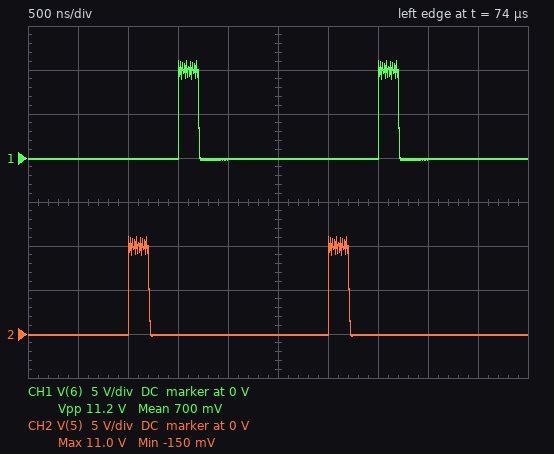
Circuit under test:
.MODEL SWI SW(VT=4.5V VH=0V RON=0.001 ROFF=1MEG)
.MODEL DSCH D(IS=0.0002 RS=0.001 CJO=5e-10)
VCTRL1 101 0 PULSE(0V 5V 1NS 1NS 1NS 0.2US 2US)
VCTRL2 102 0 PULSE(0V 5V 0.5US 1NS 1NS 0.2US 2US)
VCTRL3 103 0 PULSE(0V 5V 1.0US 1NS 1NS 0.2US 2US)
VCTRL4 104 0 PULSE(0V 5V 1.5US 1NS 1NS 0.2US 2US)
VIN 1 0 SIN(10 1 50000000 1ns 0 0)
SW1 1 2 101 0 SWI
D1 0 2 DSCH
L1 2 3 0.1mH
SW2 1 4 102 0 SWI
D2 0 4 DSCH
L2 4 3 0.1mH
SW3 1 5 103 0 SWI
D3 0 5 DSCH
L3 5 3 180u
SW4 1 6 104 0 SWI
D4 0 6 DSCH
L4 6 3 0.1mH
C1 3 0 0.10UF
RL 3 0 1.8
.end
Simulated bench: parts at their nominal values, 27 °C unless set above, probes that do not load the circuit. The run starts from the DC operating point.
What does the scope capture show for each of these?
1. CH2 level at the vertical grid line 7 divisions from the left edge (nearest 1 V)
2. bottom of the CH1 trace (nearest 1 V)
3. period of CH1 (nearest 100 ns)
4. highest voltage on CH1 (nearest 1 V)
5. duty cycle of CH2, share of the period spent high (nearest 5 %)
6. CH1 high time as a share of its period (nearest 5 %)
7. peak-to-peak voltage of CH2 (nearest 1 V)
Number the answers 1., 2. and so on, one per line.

1. 0 V
2. 0 V
3. 2.0 µs
4. 11 V
5. 10 %
6. 10 %
7. 11 V
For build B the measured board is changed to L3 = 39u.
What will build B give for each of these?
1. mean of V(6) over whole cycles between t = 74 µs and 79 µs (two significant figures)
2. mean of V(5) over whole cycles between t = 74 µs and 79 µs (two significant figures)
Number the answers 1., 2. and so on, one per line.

1. 900 mV
2. 870 mV
